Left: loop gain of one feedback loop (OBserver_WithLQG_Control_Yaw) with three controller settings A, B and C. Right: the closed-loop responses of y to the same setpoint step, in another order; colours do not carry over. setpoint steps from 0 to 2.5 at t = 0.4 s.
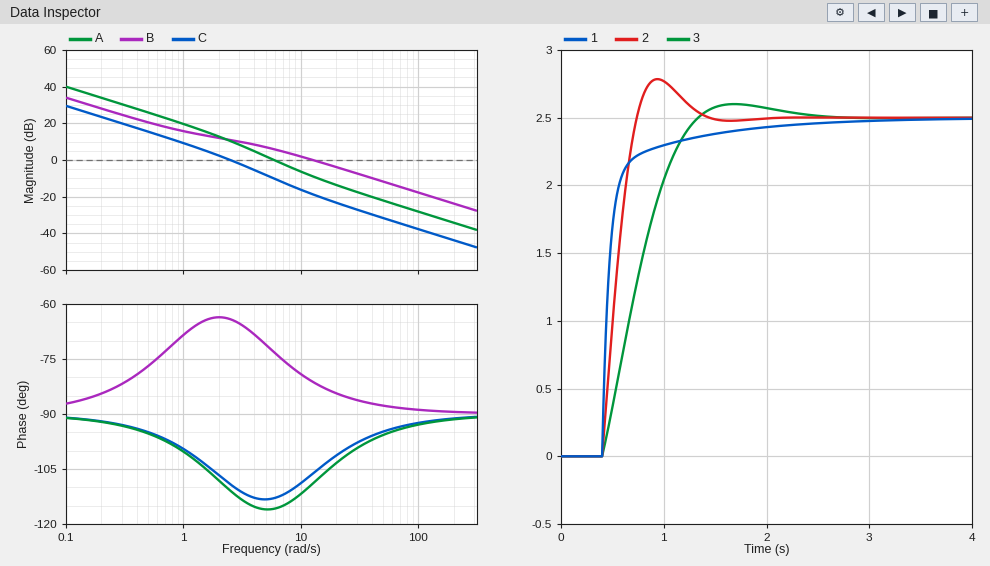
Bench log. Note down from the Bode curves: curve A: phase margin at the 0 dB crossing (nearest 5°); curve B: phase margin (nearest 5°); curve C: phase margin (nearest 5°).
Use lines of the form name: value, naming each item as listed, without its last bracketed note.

curve A: phase margin at the 0 dB crossing: 65°
curve B: phase margin: 100°
curve C: phase margin: 70°
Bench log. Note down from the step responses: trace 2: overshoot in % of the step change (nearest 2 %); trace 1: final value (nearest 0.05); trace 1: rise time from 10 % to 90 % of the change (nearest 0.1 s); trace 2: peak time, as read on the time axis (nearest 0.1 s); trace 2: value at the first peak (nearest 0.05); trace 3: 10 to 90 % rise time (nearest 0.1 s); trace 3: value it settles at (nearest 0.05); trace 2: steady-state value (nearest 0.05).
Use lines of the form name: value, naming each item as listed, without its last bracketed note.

trace 2: overshoot in % of the step change: 12 %
trace 1: final value: 2.50
trace 1: rise time from 10 % to 90 % of the change: 0.4 s
trace 2: peak time, as read on the time axis: 0.9 s
trace 2: value at the first peak: 2.80
trace 3: 10 to 90 % rise time: 0.6 s
trace 3: value it settles at: 2.50
trace 2: steady-state value: 2.50
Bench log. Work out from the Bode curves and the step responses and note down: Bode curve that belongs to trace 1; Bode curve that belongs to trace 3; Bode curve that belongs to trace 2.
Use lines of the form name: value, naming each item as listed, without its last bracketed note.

Bode curve that belongs to trace 1: B
Bode curve that belongs to trace 3: C
Bode curve that belongs to trace 2: A
